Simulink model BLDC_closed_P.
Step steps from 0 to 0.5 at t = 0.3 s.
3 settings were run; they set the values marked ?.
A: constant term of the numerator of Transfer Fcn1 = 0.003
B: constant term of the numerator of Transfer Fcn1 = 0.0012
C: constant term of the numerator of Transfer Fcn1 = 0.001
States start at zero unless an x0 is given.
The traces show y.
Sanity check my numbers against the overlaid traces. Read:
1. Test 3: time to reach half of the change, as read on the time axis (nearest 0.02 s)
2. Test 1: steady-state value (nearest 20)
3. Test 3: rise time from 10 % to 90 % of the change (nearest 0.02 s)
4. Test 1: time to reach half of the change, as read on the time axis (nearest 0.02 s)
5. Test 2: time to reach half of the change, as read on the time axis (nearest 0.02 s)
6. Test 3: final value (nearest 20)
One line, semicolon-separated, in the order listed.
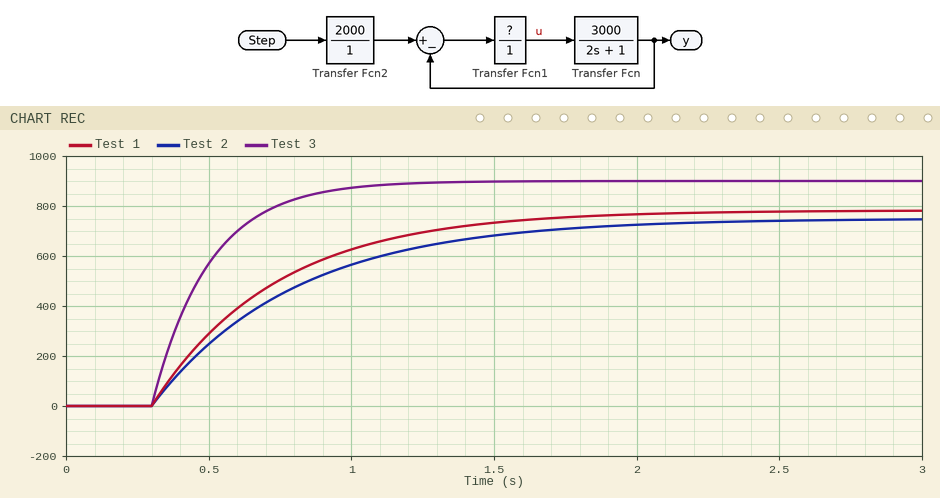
0.44 s; 780; 0.44 s; 0.60 s; 0.64 s; 900
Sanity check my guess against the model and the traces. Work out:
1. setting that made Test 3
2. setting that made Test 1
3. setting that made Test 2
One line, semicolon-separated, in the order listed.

A; B; C
